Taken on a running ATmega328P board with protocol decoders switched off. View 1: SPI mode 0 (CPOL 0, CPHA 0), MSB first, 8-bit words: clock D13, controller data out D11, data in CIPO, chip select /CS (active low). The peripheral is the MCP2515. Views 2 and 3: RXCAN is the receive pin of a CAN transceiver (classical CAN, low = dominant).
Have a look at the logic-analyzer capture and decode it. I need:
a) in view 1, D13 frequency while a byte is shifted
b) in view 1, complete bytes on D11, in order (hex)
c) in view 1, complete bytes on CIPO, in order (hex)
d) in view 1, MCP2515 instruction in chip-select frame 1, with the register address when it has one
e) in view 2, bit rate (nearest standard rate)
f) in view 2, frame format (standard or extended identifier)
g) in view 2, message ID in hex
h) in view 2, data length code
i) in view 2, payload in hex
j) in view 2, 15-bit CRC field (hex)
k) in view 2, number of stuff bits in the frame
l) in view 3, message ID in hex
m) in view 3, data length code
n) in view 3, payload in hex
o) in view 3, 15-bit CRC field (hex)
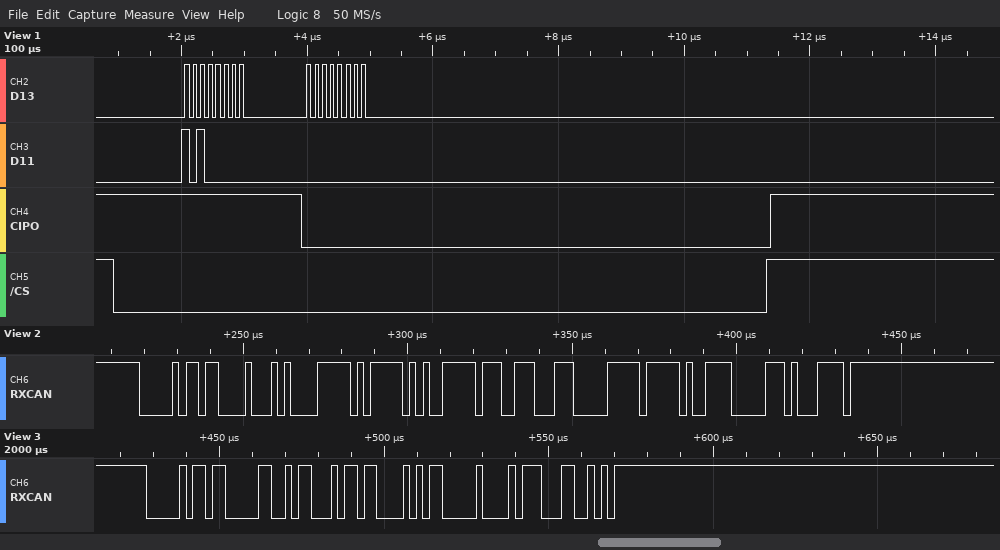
8 MHz
A0 00
FF 00
READ STATUS
500 kbit/s
standard
0x036
8
A1 FB F4 FF 38 E0 FF CF
0x0347
8
0x036
4
B1 6C 2B 00
0x2E32
